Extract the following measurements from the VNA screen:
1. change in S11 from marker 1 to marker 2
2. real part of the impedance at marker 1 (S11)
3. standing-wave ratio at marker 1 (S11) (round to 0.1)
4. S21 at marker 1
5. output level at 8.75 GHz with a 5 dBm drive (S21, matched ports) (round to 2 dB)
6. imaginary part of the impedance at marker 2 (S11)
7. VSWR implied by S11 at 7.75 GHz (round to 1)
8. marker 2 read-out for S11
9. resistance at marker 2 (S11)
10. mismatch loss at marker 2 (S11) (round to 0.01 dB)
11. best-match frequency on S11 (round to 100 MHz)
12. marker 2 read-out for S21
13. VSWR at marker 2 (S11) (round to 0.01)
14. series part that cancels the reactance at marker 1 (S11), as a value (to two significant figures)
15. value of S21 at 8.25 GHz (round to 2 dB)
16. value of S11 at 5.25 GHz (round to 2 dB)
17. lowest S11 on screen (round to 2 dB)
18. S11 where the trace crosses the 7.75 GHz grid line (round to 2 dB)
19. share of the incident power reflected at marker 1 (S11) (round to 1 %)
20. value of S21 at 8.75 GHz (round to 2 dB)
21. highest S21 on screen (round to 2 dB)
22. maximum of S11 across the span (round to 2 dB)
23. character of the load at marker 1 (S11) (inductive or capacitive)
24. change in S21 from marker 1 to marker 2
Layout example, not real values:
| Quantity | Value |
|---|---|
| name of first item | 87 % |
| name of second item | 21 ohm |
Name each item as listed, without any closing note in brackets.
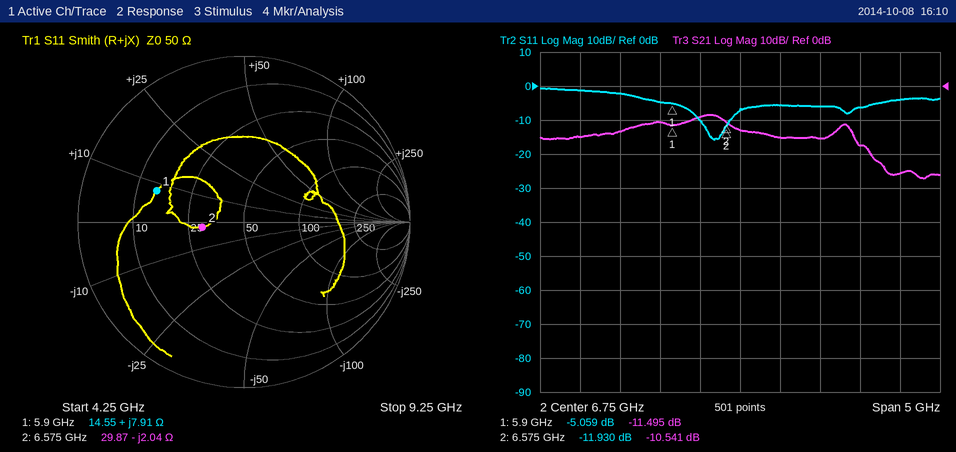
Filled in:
| Quantity | Value |
|---|---|
| change in S11 from marker 1 to marker 2 | -6.871 dB |
| real part of the impedance at marker 1 | 14.55 Ω |
| standing-wave ratio at marker 1 (S11) | 3.5 |
| S21 at marker 1 | -11.495 dB |
| output level at 8.75 GHz with a 5 dBm drive (S21, matched ports) | -20 dBm |
| imaginary part of the impedance at marker 2 | -2.04 Ω |
| VSWR implied by S11 at 7.75 GHz | 3 |
| marker 2 read-out for S11 | -11.930 dB |
| resistance at marker 2 | 29.87 Ω |
| mismatch loss at marker 2 (S11) | 0.29 dB |
| best-match frequency on S11 | 6.4 GHz |
| marker 2 read-out for S21 | -10.541 dB |
| VSWR at marker 2 (S11) | 1.68 |
| series part that cancels the reactance at marker 1 (S11), as a value | 3.4 pF |
| value of S21 at 8.25 GHz | -18 dB |
| value of S11 at 5.25 GHz | -2 dB |
| lowest S11 on screen | -16 dB |
| S11 where the trace crosses the 7.75 GHz grid line | -6 dB |
| share of the incident power reflected at marker 1 (S11) | 31 % |
| value of S21 at 8.75 GHz | -26 dB |
| highest S21 on screen | -8 dB |
| maximum of S11 across the span | 0 dB |
| character of the load at marker 1 (S11) | inductive |
| change in S21 from marker 1 to marker 2 | 0.954 dB |
